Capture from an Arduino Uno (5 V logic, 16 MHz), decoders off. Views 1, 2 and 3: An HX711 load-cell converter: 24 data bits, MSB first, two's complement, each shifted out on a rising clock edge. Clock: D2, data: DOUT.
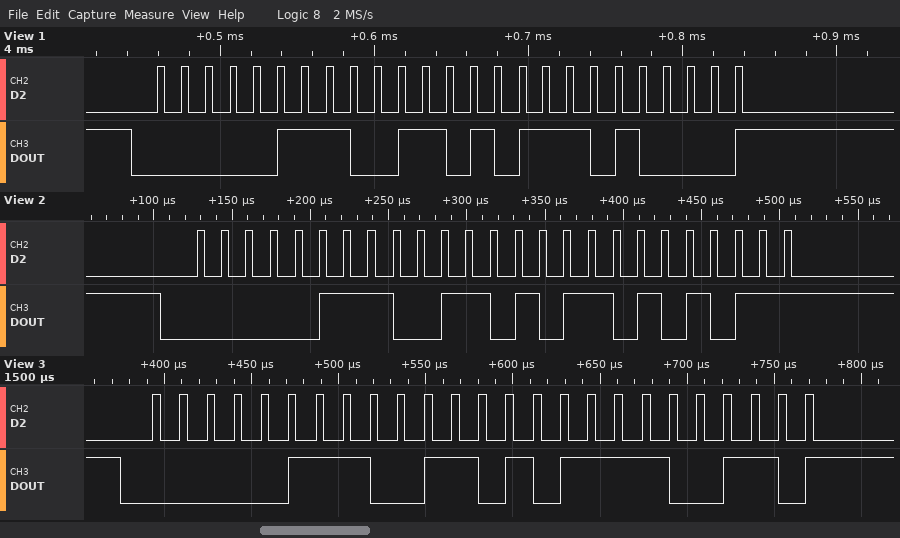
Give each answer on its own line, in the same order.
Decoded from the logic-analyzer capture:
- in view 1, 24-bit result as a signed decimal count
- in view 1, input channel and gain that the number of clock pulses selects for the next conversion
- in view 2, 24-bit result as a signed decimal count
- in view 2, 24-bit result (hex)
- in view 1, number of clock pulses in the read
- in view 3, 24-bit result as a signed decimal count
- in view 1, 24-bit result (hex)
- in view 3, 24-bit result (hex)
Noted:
472528
channel A, gain 128
472491
0x0735AB
25
472550
0x0735D0
0x0735E6
